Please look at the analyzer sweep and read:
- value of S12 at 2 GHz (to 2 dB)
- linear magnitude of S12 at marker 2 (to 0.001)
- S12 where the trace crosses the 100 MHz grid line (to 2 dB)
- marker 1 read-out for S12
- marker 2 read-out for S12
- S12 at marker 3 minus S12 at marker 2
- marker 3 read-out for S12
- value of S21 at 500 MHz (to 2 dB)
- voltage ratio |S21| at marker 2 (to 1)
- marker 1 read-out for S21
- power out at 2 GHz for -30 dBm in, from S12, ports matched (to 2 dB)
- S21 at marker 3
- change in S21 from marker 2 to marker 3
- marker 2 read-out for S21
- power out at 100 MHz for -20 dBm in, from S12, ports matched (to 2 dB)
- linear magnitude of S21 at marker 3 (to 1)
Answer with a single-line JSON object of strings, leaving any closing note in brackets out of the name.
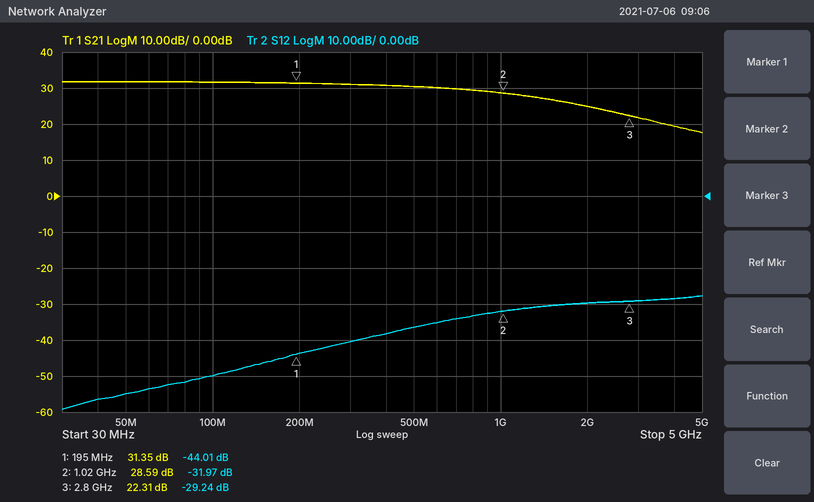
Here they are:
{"value of S12 at 2 GHz": "-30 dB", "linear magnitude of S12 at marker 2": "0.025", "S12 where the trace crosses the 100 MHz grid line": "-50 dB", "marker 1 read-out for S12": "-44.01 dB", "marker 2 read-out for S12": "-31.97 dB", "S12 at marker 3 minus S12 at marker 2": "2.73 dB", "marker 3 read-out for S12": "-29.24 dB", "value of S21 at 500 MHz": "30 dB", "voltage ratio |S21| at marker 2": "27", "marker 1 read-out for S21": "31.35 dB", "power out at 2 GHz for -30 dBm in, from S12, ports matched": "-60 dBm", "S21 at marker 3": "22.31 dB", "change in S21 from marker 2 to marker 3": "-6.28 dB", "marker 2 read-out for S21": "28.59 dB", "power out at 100 MHz for -20 dBm in, from S12, ports matched": "-70 dBm", "linear magnitude of S21 at marker 3": "13"}
